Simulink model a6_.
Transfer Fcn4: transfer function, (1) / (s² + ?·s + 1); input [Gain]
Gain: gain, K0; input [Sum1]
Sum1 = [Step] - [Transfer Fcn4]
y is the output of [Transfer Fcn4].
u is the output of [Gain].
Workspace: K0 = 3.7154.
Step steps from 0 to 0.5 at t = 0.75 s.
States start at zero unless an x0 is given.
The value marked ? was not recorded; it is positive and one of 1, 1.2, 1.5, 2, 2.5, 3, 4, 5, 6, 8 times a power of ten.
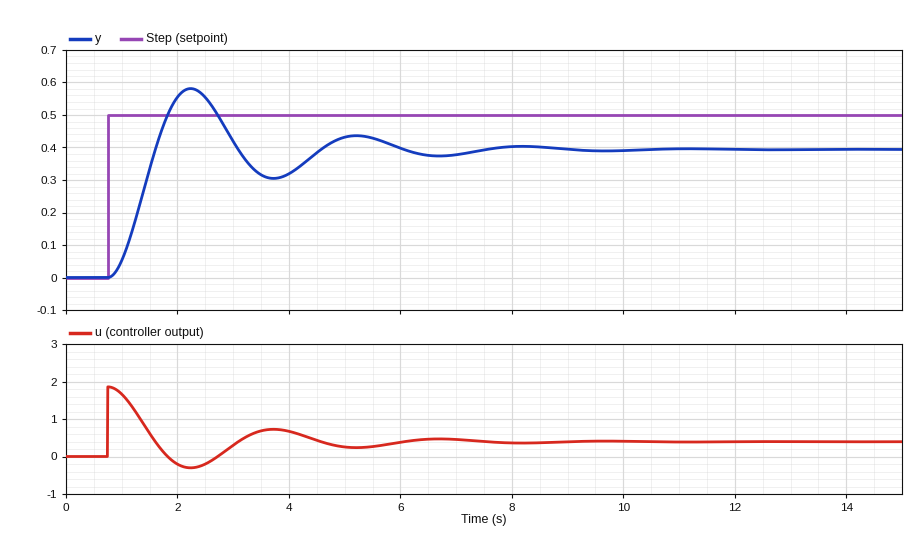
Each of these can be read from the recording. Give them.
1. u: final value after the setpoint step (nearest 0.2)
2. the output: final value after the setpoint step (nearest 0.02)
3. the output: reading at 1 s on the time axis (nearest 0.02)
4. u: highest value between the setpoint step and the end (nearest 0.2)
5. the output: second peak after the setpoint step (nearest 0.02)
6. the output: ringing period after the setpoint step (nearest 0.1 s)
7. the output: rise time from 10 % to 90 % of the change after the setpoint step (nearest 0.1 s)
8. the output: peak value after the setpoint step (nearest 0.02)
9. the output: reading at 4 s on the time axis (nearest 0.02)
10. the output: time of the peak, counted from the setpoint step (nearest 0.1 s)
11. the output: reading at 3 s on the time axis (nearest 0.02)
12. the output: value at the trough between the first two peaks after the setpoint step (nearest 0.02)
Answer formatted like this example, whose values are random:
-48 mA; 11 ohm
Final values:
0.4; 0.40; 0.06; 1.8; 0.44; 3.0 s; 0.6 s; 0.58; 0.32; 1.5 s; 0.42; 0.30
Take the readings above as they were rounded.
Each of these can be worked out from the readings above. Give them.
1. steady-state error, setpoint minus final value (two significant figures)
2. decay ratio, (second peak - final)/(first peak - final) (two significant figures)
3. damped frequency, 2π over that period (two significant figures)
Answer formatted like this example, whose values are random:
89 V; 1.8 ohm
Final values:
0.10; 0.22; 2.1 rad/s
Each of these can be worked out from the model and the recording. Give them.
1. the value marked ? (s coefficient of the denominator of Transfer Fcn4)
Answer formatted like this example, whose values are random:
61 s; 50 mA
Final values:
1
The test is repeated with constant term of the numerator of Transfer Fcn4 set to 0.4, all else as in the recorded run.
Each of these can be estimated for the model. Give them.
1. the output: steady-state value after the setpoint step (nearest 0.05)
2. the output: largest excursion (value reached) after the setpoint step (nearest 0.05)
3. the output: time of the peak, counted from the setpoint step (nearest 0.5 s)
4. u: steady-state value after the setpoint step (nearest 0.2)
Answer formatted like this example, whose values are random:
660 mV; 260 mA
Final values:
0.30; 0.40; 2.0 s; 0.8
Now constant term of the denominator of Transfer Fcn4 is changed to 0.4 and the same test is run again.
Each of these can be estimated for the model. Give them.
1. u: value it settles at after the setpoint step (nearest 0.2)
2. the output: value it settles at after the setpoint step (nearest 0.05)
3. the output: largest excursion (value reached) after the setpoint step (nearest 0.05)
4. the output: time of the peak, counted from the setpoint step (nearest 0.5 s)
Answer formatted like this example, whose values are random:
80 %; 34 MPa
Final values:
0.2; 0.45; 0.65; 1.5 s
